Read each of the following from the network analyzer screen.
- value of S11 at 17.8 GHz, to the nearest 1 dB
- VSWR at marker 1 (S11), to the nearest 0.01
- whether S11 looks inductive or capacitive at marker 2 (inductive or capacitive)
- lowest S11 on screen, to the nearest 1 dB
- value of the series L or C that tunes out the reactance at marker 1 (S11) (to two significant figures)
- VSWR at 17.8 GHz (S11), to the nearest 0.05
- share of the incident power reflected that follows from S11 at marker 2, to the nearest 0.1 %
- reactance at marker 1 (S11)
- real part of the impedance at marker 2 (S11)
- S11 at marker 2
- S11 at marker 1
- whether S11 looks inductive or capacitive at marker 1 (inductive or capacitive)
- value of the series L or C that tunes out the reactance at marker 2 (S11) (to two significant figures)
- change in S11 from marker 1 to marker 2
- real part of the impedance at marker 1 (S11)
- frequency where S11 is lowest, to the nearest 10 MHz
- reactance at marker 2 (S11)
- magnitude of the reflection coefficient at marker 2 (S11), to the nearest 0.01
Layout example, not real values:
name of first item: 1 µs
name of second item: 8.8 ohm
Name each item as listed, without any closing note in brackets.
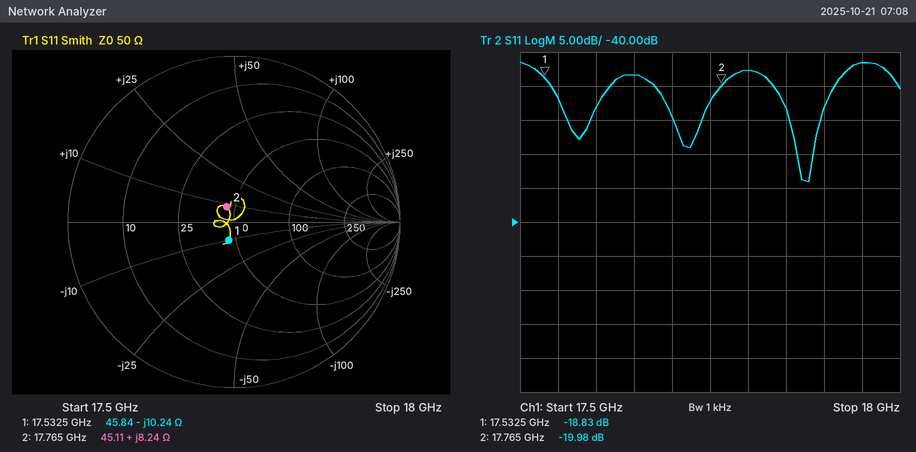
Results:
value of S11 at 17.8 GHz, to the nearest 1 dB: -18 dB
VSWR at marker 1 (S11), to the nearest 0.01: 1.26
whether S11 looks inductive or capacitive at marker 2: inductive
lowest S11 on screen, to the nearest 1 dB: -34 dB
value of the series L or C that tunes out the reactance at marker 1 (S11): 93 pH
VSWR at 17.8 GHz (S11), to the nearest 0.05: 1.30
share of the incident power reflected that follows from S11 at marker 2, to the nearest 0.1 %: 1.0 %
reactance at marker 1: -10.24 Ω
real part of the impedance at marker 2: 45.11 Ω
S11 at marker 2: -19.98 dB
S11 at marker 1: -18.83 dB
whether S11 looks inductive or capacitive at marker 1: capacitive
value of the series L or C that tunes out the reactance at marker 2 (S11): 1.1 pF
change in S11 from marker 1 to marker 2: -1.15 dB
real part of the impedance at marker 1: 45.84 Ω
frequency where S11 is lowest, to the nearest 10 MHz: 17.88 GHz
reactance at marker 2: +8.24 Ω
magnitude of the reflection coefficient at marker 2 (S11), to the nearest 0.01: 0.10
